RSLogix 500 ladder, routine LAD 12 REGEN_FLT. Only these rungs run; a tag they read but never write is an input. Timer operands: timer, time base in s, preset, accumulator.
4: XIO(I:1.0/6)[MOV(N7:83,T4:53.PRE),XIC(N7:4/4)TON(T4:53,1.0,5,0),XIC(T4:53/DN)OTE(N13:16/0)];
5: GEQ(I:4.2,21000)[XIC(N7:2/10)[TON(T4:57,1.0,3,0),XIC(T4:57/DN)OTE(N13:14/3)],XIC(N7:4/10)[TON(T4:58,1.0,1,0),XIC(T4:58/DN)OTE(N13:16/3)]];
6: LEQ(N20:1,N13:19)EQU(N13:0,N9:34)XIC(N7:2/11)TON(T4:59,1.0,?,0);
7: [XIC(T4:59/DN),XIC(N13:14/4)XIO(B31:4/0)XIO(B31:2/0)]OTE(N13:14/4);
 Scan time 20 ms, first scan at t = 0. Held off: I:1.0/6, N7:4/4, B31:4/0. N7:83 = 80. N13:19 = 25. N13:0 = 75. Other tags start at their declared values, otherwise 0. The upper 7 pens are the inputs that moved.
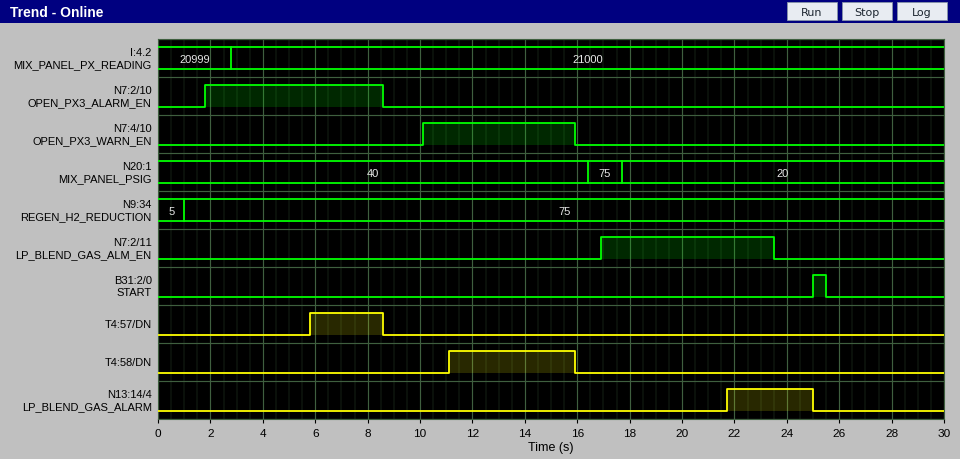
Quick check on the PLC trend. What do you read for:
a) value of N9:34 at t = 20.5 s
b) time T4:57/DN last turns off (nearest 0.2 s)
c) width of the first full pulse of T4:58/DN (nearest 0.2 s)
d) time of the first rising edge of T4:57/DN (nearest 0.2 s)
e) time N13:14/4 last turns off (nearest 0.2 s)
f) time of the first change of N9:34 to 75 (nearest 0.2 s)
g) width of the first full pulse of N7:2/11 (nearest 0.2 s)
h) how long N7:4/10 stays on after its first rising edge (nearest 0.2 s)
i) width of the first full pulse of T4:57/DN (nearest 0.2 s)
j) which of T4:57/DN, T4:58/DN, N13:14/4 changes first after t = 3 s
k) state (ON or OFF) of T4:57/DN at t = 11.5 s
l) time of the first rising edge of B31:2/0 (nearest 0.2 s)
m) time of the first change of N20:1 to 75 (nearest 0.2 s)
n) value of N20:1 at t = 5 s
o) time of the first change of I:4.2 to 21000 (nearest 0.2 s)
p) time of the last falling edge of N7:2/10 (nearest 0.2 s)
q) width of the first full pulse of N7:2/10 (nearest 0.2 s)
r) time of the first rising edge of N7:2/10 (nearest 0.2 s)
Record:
75
8.6 s
4.8 s
5.8 s
25.0 s
1.0 s
6.6 s
5.8 s
2.8 s
T4:57/DN
OFF
25.0 s
16.4 s
40
2.8 s
8.6 s
6.8 s
1.8 s
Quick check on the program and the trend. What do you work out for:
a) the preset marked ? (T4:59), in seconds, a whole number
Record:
4 s
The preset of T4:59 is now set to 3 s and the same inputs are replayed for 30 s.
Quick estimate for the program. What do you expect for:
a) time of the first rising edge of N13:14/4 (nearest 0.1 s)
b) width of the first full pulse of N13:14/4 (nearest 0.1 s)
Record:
20.7 s
4.3 s
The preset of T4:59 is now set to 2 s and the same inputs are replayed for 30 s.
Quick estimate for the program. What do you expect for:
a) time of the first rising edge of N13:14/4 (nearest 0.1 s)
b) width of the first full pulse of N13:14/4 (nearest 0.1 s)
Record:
19.7 s
5.3 s
